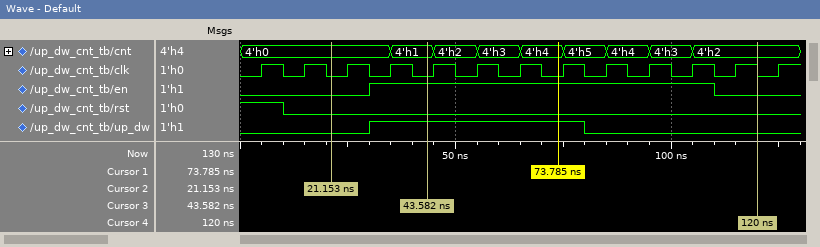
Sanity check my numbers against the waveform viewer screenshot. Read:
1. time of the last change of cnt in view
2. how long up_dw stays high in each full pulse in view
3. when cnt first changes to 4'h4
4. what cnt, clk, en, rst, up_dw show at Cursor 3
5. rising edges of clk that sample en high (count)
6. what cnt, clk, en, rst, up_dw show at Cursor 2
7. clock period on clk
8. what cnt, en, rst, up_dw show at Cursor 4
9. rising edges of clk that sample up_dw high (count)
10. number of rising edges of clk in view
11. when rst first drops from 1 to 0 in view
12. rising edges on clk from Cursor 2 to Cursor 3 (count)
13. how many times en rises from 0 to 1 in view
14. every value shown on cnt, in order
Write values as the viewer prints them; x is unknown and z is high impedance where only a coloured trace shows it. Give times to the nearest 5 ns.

105 ns
50 ns
65 ns
cnt=4'h1, clk=0, en=1, rst=0, up_dw=1
8
cnt=4'h0, clk=0, en=0, rst=0, up_dw=0
10 ns
cnt=4'h2, en=0, rst=0, up_dw=0
5
13
10 ns
2
1
4'h0, 4'h1, 4'h2, 4'h3, 4'h4, 4'h5, 4'h4, 4'h3, 4'h2
